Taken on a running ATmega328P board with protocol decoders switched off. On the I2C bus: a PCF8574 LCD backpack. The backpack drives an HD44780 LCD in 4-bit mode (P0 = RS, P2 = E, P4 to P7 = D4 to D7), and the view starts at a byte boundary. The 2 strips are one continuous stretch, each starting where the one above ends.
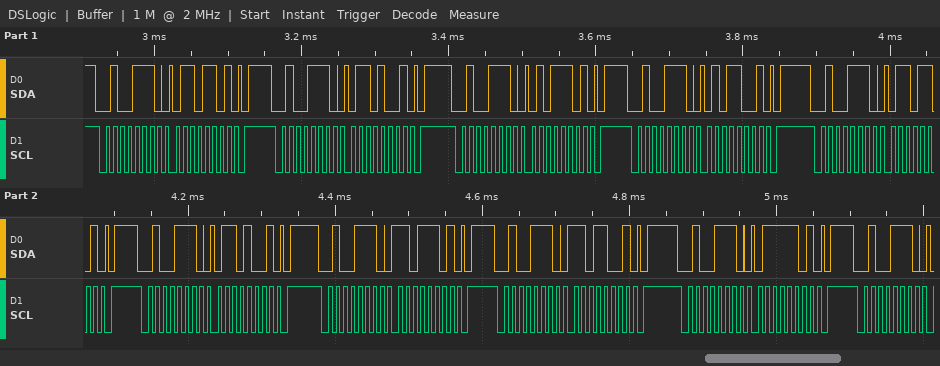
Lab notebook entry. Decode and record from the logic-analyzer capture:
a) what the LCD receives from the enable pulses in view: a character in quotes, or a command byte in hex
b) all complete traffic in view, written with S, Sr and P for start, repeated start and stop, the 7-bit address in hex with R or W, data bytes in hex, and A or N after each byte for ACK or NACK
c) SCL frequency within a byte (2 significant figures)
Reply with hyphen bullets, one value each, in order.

- 'e' 'm'
- S 27W A 6D A P S 27W A 69 A P S 27W A 5D A P S 27W A 59 A P S 27W A 6D A P S 27W A 69 A P S 27W A DD A P S 27W A D9 A P S 27W A 7D A P S 27W A
- 100 kHz
